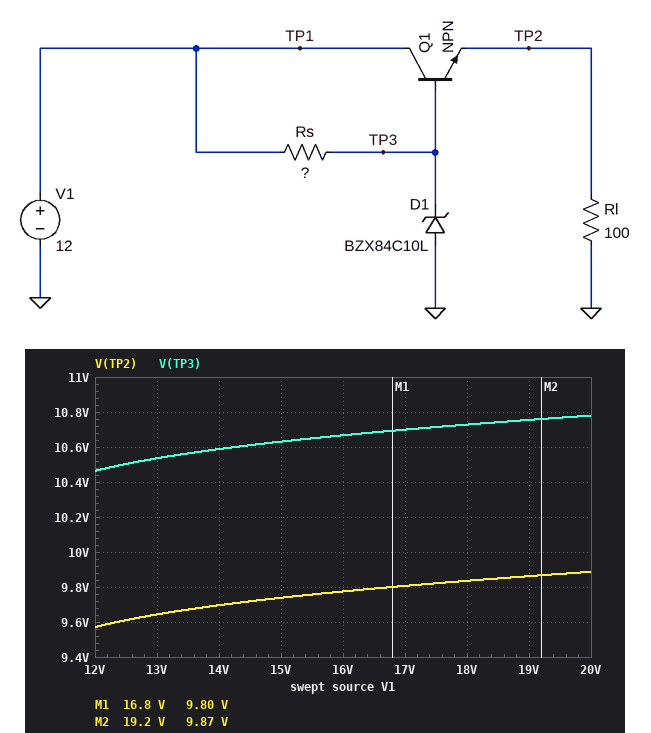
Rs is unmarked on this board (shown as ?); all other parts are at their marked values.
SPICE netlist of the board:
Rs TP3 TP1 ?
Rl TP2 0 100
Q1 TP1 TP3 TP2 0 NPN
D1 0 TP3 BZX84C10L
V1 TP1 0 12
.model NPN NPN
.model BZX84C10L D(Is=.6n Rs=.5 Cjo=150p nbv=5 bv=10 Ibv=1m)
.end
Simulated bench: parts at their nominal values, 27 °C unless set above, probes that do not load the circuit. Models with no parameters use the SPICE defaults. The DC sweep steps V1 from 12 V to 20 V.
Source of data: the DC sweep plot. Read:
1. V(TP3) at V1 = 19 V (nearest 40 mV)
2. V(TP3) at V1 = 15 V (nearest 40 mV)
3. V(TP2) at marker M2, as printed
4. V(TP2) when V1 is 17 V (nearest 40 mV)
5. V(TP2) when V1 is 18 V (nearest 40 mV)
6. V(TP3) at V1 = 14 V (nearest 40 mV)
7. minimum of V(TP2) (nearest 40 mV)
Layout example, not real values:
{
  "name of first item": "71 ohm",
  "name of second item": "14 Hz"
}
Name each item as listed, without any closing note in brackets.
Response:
{
  "V(TP3) at V1 = 19 V": "10.76 V",
  "V(TP3) at V1 = 15 V": "10.64 V",
  "V(TP2) at marker M2, as printed": "9.87 V",
  "V(TP2) when V1 is 17 V": "9.80 V",
  "V(TP2) when V1 is 18 V": "9.84 V",
  "V(TP3) at V1 = 14 V": "10.60 V",
  "minimum of V(TP2)": "9.56 V"
}
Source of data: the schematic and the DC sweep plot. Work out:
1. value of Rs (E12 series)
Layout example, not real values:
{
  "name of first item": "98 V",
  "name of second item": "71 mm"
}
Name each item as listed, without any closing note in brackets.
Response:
{
  "value of Rs": "47 Ω"
}
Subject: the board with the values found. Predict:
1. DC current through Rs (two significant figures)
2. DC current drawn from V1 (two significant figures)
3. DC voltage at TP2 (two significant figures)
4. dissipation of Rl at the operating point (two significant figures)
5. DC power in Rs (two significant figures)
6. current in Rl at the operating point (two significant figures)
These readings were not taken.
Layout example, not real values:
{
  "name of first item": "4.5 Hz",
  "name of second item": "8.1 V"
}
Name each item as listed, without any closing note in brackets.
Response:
{
  "DC current through Rs": "33 mA",
  "DC current drawn from V1": "130 mA",
  "DC voltage at TP2": "9.6 V",
  "dissipation of Rl at the operating point": "920 mW",
  "DC power in Rs": "50 mW",
  "current in Rl at the operating point": "96 mA"
}
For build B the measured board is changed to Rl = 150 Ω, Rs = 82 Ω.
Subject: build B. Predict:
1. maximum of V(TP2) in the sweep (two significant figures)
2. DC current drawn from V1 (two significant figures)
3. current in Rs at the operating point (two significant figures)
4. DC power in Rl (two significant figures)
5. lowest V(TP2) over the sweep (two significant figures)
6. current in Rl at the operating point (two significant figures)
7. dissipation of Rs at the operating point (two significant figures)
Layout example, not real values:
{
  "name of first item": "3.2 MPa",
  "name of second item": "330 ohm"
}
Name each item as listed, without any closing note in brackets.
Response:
{
  "maximum of V(TP2) in the sweep": "9.8 V",
  "DC current drawn from V1": "82 mA",
  "current in Rs at the operating point": "20 mA",
  "DC power in Rl": "600 mW",
  "lowest V(TP2) over the sweep": "9.5 V",
  "current in Rl at the operating point": "63 mA",
  "dissipation of Rs at the operating point": "32 mW"
}
